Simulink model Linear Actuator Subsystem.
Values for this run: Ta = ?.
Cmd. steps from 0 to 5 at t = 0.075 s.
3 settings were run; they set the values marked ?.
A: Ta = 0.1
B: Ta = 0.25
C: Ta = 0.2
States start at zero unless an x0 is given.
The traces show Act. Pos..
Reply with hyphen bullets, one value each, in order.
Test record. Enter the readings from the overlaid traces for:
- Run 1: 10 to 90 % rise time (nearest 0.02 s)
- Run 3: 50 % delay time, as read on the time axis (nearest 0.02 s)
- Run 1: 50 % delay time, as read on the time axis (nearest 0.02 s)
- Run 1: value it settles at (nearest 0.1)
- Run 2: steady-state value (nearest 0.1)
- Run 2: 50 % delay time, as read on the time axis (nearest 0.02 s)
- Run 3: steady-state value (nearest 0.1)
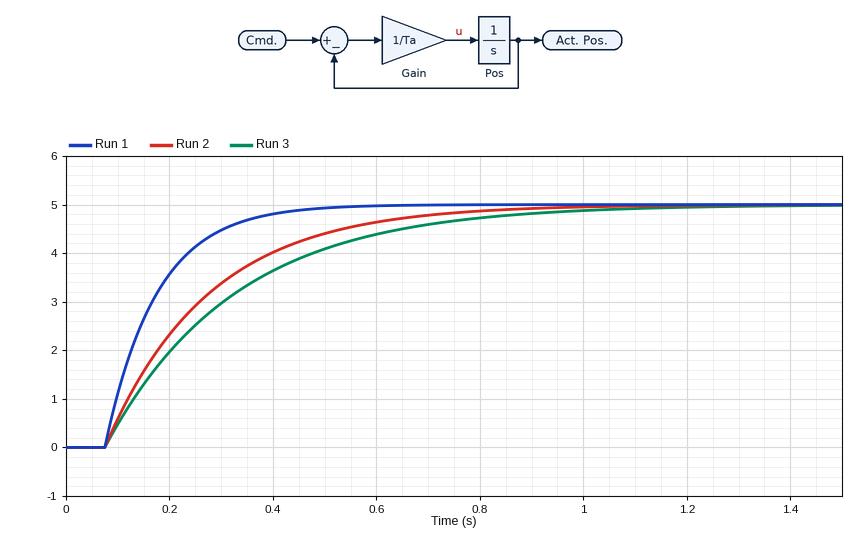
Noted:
- 0.22 s
- 0.24 s
- 0.14 s
- 5.0
- 5.0
- 0.22 s
- 5.0
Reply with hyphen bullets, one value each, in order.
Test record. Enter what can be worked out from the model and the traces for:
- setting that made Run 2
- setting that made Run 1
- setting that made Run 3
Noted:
- C
- A
- B
